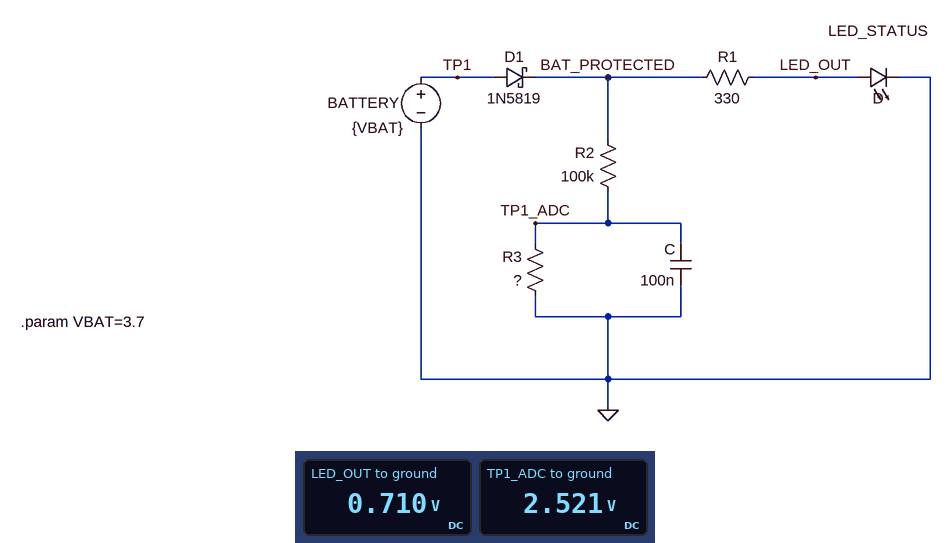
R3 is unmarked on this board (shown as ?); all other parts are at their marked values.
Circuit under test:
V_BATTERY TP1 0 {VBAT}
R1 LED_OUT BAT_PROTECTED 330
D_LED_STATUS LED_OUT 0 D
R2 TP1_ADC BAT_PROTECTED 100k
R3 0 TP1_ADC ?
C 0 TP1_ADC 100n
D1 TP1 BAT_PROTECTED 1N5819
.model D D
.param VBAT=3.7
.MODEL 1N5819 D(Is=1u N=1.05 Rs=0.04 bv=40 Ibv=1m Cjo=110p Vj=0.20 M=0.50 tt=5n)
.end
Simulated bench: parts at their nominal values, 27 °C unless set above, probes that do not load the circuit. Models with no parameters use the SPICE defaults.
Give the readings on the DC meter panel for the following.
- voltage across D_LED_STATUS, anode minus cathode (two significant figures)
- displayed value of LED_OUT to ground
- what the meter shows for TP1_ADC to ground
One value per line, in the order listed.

710 mV
0.710 V
2.521 V
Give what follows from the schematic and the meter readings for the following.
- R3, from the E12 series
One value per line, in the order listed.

270 kΩ
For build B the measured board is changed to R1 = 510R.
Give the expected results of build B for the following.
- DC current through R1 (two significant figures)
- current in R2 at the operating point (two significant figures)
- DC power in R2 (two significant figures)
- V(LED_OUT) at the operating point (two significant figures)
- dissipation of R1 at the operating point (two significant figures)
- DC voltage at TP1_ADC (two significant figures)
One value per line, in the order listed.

5.4 mA
9.4 µA
8.8 µW
700 mV
15 mW
2.5 V
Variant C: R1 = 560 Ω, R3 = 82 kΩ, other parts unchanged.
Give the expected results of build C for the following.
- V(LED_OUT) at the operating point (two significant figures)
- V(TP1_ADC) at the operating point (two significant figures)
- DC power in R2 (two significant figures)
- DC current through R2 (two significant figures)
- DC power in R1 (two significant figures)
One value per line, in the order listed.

700 mV
1.6 V
36 µW
19 µA
14 mW
